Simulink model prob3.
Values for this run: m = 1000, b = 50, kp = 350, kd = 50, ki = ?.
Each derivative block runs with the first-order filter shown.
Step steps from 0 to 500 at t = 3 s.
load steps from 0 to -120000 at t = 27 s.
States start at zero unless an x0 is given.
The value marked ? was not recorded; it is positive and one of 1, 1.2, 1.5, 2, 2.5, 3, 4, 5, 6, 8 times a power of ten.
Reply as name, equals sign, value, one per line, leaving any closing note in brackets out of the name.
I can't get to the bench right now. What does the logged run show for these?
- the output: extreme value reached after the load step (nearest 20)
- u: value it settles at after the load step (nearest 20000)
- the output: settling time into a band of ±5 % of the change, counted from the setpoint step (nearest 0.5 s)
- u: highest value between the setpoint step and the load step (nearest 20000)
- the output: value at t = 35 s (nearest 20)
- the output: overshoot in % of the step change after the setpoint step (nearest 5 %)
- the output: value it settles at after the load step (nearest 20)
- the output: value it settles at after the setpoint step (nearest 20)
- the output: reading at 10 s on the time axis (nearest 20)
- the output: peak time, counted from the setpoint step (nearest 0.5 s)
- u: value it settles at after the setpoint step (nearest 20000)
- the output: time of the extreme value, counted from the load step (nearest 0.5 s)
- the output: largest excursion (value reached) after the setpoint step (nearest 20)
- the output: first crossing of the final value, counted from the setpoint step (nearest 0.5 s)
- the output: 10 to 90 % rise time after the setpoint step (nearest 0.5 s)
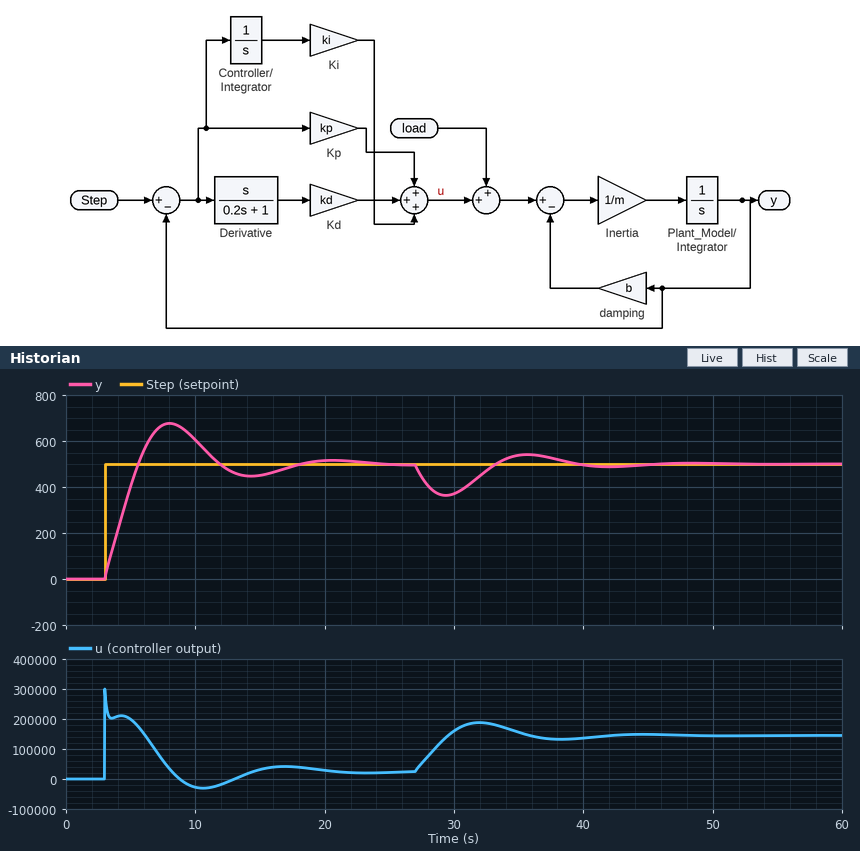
the output: extreme value reached after the load step = 360
u: value it settles at after the load step = 140000
the output: settling time into a band of ±5 % of the change, counted from the setpoint step = 13.5 s
u: highest value between the setpoint step and the load step = 300000
the output: value at t = 35 s = 540
the output: overshoot in % of the step change after the setpoint step = 35 %
the output: value it settles at after the load step = 500
the output: value it settles at after the setpoint step = 500
the output: reading at 10 s on the time axis = 600
the output: peak time, counted from the setpoint step = 5.0 s
u: value it settles at after the setpoint step = 20000
the output: time of the extreme value, counted from the load step = 2.5 s
the output: largest excursion (value reached) after the setpoint step = 680
the output: first crossing of the final value, counted from the setpoint step = 2.5 s
the output: 10 to 90 % rise time after the setpoint step = 2.0 s
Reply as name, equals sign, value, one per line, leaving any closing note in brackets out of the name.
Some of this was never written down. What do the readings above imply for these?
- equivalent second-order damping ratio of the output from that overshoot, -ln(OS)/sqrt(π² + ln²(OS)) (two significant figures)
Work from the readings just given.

equivalent second-order damping ratio of the output from that overshoot, -ln(OS)/sqrt(π² + ln²(OS)) = 0.32
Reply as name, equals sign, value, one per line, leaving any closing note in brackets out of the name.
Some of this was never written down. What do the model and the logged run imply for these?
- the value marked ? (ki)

the value marked ? = 300
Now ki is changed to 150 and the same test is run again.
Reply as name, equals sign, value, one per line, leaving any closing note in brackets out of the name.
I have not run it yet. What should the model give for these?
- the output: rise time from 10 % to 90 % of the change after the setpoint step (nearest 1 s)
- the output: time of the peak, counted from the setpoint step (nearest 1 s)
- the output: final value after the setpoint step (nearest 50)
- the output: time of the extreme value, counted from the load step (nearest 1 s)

the output: rise time from 10 % to 90 % of the change after the setpoint step = 3 s
the output: time of the peak, counted from the setpoint step = 7 s
the output: final value after the setpoint step = 500
the output: time of the extreme value, counted from the load step = 3 s
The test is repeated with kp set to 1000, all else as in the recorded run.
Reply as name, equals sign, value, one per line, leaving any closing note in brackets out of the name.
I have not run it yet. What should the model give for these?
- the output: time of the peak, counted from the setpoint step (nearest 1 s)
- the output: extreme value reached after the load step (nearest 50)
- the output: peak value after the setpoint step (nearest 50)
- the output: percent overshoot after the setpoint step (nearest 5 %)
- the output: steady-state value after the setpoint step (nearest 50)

the output: time of the peak, counted from the setpoint step = 4 s
the output: extreme value reached after the load step = 400
the output: peak value after the setpoint step = 550
the output: percent overshoot after the setpoint step = 10 %
the output: steady-state value after the setpoint step = 500
